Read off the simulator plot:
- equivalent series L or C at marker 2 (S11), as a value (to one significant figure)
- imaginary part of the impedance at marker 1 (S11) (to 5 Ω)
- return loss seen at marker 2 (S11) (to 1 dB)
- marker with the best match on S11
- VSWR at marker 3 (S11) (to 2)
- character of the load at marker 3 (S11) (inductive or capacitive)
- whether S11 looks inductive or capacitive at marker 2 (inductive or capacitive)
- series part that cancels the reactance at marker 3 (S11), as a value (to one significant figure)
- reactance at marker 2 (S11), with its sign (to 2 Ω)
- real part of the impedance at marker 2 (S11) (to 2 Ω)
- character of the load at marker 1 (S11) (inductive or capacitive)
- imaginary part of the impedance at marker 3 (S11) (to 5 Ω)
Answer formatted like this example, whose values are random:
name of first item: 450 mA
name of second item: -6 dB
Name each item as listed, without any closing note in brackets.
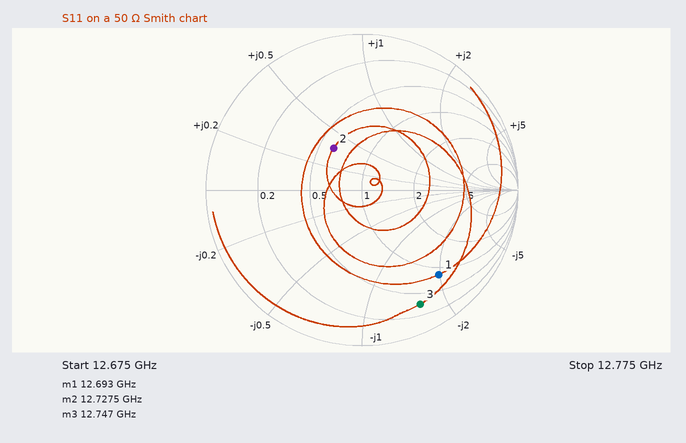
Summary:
equivalent series L or C at marker 2 (S11), as a value: 200 pH
imaginary part of the impedance at marker 1 (S11): -100 Ω
return loss seen at marker 2 (S11): 10 dB
marker with the best match on S11: marker 2
VSWR at marker 3 (S11): 10
character of the load at marker 3 (S11): capacitive
whether S11 looks inductive or capacitive at marker 2: inductive
series part that cancels the reactance at marker 3 (S11), as a value: 1.0 nH
reactance at marker 2 (S11), with its sign: +18 Ω
real part of the impedance at marker 2 (S11): 30 Ω
character of the load at marker 1 (S11): capacitive
imaginary part of the impedance at marker 3 (S11): -80 Ω
